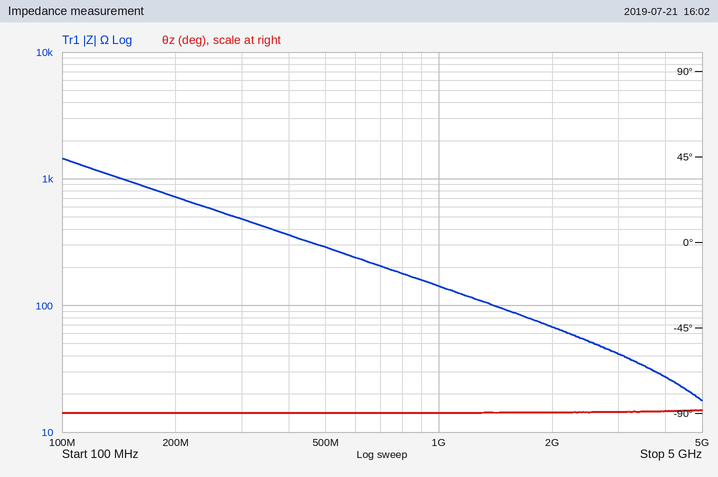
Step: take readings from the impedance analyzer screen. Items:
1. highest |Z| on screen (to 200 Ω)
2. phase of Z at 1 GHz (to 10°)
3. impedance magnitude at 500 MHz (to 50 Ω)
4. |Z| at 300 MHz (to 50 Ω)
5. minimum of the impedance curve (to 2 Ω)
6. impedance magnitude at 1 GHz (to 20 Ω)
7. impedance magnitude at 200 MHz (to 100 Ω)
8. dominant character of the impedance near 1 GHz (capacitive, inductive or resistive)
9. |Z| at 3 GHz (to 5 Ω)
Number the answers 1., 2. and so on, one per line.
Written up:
1. 1.4 kΩ
2. -90°
3. 300 Ω
4. 500 Ω
5. 18 Ω
6. 140 Ω
7. 700 Ω
8. capacitive
9. 40 Ω
